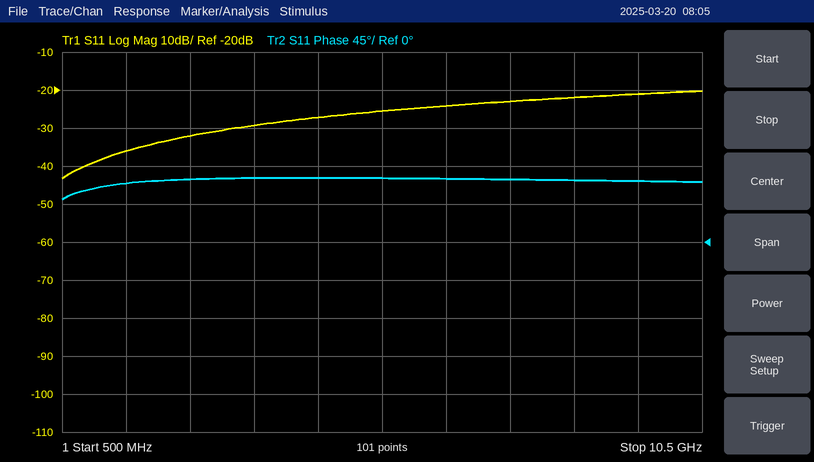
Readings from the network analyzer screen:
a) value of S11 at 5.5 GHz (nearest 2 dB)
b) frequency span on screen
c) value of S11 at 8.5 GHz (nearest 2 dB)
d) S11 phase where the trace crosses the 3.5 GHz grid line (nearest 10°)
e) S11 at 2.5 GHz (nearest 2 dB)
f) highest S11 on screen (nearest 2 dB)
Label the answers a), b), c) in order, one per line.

a) -26 dB
b) 10 GHz
c) -22 dB
d) 80°
e) -32 dB
f) -20 dB
